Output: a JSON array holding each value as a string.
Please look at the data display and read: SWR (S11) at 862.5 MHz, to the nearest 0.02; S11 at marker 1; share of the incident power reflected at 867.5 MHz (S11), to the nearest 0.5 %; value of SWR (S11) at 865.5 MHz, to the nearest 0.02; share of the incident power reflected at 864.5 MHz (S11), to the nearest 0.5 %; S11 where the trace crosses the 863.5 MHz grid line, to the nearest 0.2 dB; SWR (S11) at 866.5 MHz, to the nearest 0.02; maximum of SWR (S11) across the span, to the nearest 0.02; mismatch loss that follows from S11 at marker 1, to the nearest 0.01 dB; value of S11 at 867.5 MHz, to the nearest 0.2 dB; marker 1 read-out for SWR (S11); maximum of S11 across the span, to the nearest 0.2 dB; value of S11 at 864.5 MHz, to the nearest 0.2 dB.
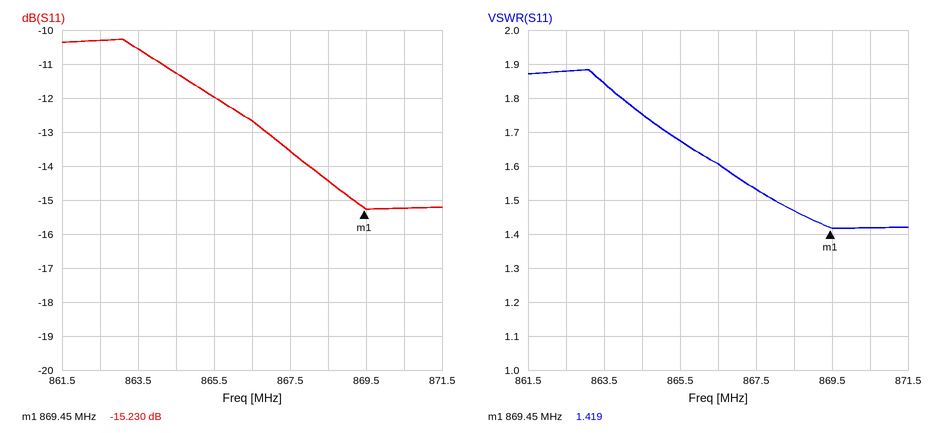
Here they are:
["1.88", "-15.230 dB", "4.5 %", "1.68", "7.5 %", "-10.6 dB", "1.60", "1.88", "0.13 dB", "-13.6 dB", "1.419", "-10.2 dB", "-11.2 dB"]
